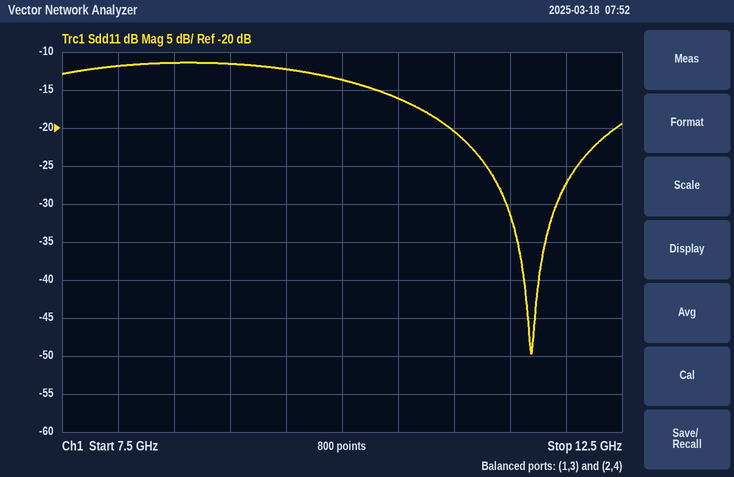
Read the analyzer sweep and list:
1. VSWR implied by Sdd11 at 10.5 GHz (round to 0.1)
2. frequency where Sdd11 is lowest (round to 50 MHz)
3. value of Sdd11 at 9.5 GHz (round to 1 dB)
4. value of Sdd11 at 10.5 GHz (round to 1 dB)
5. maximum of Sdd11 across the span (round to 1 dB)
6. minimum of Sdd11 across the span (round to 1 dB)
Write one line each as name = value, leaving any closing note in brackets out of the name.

VSWR implied by Sdd11 at 10.5 GHz = 1.4
frequency where Sdd11 is lowest = 11.70 GHz
value of Sdd11 at 9.5 GHz = -12 dB
value of Sdd11 at 10.5 GHz = -16 dB
maximum of Sdd11 across the span = -11 dB
minimum of Sdd11 across the span = -50 dB
